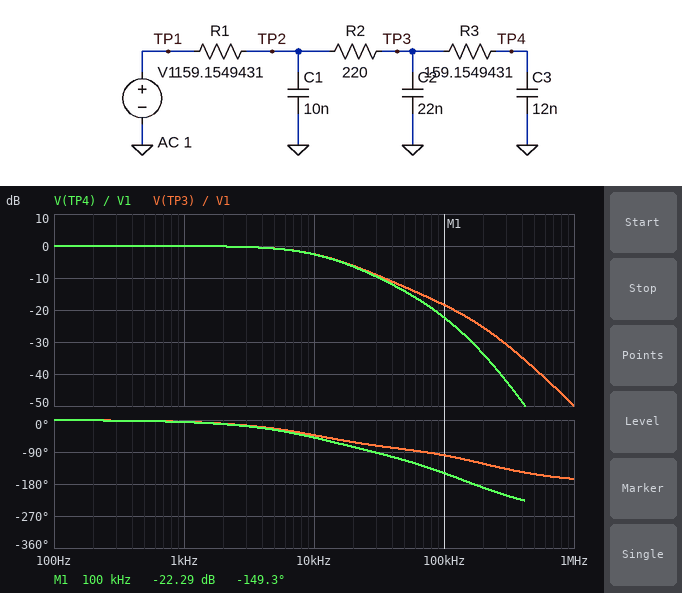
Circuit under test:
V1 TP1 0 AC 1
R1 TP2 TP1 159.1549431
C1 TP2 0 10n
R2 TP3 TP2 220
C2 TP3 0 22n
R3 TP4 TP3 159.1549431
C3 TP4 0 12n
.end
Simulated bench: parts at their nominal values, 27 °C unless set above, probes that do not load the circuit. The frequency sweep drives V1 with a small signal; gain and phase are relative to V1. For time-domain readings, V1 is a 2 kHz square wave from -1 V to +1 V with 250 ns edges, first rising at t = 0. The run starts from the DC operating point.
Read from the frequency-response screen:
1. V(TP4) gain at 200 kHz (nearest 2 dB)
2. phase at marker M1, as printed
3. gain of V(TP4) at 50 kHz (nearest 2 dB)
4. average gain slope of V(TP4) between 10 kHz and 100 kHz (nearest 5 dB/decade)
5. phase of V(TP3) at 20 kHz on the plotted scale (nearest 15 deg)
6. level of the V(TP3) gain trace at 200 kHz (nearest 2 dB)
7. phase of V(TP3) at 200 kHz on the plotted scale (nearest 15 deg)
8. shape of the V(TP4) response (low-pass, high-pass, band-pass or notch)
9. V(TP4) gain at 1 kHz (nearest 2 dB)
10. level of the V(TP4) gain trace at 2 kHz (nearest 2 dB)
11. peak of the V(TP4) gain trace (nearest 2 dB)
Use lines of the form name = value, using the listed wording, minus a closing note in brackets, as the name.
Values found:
V(TP4) gain at 200 kHz = -34 dB
phase at marker M1, as printed = -149.3 deg
gain of V(TP4) at 50 kHz = -14 dB
average gain slope of V(TP4) between 10 kHz and 100 kHz = -20 dB/decade
phase of V(TP3) at 20 kHz on the plotted scale = -60 deg
level of the V(TP3) gain trace at 200 kHz = -26 dB
phase of V(TP3) at 200 kHz on the plotted scale = -120 deg
shape of the V(TP4) response = low-pass
V(TP4) gain at 1 kHz = 0 dB
level of the V(TP4) gain trace at 2 kHz = 0 dB
peak of the V(TP4) gain trace = 0 dB
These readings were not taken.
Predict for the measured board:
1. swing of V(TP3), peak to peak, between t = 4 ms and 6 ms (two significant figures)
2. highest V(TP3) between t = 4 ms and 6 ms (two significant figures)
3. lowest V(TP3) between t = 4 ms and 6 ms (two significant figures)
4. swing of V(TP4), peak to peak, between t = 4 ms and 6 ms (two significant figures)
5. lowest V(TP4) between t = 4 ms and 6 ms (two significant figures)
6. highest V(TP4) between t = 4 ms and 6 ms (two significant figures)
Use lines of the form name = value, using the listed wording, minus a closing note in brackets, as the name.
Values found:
swing of V(TP3), peak to peak, between t = 4 ms and 6 ms = 2.0 V
highest V(TP3) between t = 4 ms and 6 ms = 1.0 V
lowest V(TP3) between t = 4 ms and 6 ms = -1.0 V
swing of V(TP4), peak to peak, between t = 4 ms and 6 ms = 2.0 V
lowest V(TP4) between t = 4 ms and 6 ms = -1.0 V
highest V(TP4) between t = 4 ms and 6 ms = 1.0 V
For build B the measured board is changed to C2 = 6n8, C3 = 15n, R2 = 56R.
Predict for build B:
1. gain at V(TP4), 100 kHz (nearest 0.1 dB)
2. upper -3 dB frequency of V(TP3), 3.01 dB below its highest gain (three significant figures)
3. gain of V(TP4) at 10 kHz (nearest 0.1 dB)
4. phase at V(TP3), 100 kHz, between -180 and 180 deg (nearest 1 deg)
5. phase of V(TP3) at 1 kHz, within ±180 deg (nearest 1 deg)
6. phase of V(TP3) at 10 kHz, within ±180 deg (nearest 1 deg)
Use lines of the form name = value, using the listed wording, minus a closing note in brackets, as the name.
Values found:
gain at V(TP4), 100 kHz = -15.2 dB
upper -3 dB frequency of V(TP3), 3.01 dB below its highest gain = 23.3 kHz
gain of V(TP4) at 10 kHz = -0.9 dB
phase at V(TP3), 100 kHz, between -180 and 180 deg = -61 deg
phase of V(TP3) at 1 kHz, within ±180 deg = -2 deg
phase of V(TP3) at 10 kHz, within ±180 deg = -21 deg
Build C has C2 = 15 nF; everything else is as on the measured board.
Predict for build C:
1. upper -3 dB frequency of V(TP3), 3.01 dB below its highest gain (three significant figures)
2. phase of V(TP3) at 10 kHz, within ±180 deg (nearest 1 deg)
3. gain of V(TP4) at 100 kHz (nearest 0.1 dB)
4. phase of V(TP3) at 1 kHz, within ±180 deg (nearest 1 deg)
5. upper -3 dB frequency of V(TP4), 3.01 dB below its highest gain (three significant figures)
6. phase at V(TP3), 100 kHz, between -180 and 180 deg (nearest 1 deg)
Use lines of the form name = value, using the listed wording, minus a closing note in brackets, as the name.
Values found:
upper -3 dB frequency of V(TP3), 3.01 dB below its highest gain = 13.6 kHz
phase of V(TP3) at 10 kHz, within ±180 deg = -37 deg
gain of V(TP4) at 100 kHz = -20.2 dB
phase of V(TP3) at 1 kHz, within ±180 deg = -4 deg
upper -3 dB frequency of V(TP4), 3.01 dB below its highest gain = 13.3 kHz
phase at V(TP3), 100 kHz, between -180 and 180 deg = -93 deg
